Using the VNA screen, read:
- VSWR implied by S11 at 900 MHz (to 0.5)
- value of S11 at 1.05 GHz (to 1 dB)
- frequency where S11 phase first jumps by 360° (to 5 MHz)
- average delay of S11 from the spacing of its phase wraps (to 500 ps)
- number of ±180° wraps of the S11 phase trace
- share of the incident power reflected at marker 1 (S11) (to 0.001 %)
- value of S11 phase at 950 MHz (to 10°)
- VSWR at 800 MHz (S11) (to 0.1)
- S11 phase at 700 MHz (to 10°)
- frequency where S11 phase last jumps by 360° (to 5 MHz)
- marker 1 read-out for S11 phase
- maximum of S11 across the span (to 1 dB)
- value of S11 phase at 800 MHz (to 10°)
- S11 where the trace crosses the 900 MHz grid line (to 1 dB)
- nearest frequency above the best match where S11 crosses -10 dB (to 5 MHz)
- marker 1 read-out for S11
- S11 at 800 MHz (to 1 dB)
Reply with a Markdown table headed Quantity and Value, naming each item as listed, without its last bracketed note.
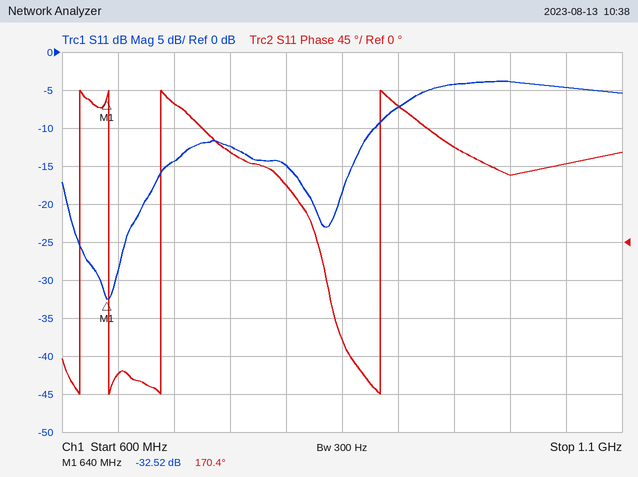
| Quantity | Value |
|---|---|
| VSWR implied by S11 at 900 MHz | 2.5 |
| value of S11 at 1.05 GHz | -5 dB |
| frequency where S11 phase first jumps by 360° | 615 MHz |
| average delay of S11 from the spacing of its phase wraps | 11.0 ns |
| number of ±180° wraps of the S11 phase trace | 4 |
| share of the incident power reflected at marker 1 (S11) | 0.056 % |
| value of S11 phase at 950 MHz | 110° |
| VSWR at 800 MHz (S11) | 1.4 |
| S11 phase at 700 MHz | 160° |
| frequency where S11 phase last jumps by 360° | 885 MHz |
| marker 1 read-out for S11 phase | 170.4° |
| maximum of S11 across the span | -4 dB |
| value of S11 phase at 800 MHz | 70° |
| S11 where the trace crosses the 900 MHz grid line | -7 dB |
| nearest frequency above the best match where S11 crosses -10 dB | 880 MHz |
| marker 1 read-out for S11 | -32.52 dB |
| S11 at 800 MHz | -15 dB |
